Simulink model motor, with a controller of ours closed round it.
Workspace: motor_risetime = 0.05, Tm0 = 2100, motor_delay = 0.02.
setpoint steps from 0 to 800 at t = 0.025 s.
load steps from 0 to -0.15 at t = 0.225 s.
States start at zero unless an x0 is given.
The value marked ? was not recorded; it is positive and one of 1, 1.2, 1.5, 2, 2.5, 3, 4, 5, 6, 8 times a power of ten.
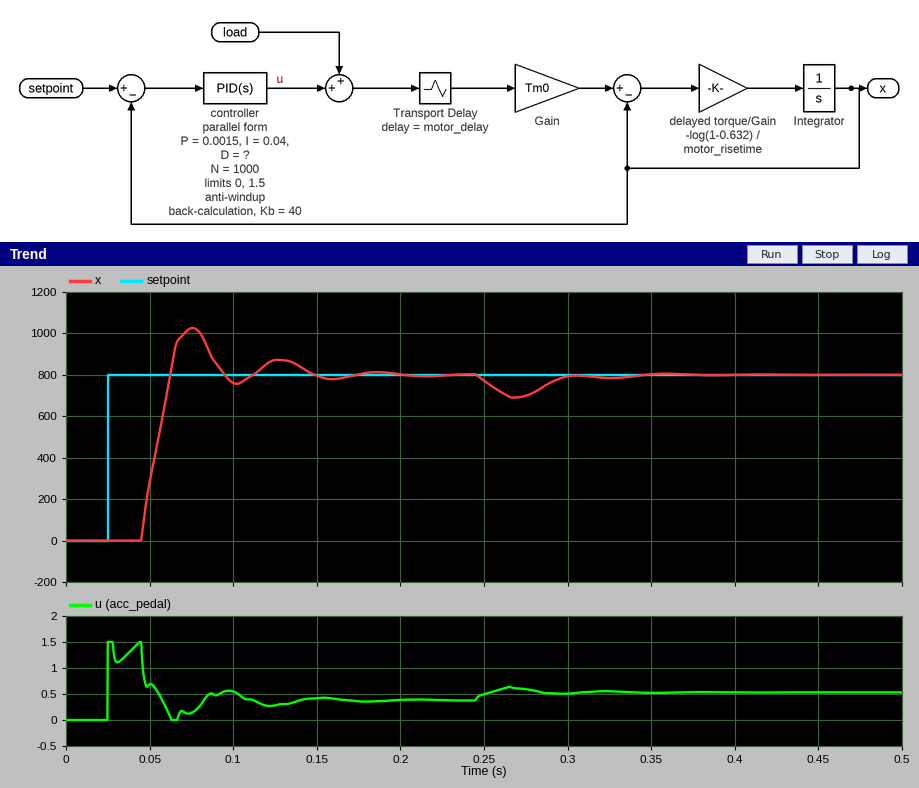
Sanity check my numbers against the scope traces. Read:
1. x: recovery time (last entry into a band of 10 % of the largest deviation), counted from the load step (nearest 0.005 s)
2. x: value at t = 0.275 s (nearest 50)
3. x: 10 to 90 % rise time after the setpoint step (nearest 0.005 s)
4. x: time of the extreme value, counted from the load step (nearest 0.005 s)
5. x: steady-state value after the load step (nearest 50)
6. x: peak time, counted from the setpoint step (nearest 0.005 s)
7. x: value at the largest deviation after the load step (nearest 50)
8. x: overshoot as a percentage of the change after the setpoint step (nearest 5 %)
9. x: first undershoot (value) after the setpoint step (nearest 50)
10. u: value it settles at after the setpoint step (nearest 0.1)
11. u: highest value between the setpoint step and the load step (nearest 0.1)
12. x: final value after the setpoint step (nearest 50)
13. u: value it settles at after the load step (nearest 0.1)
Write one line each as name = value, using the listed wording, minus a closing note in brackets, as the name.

x: recovery time (last entry into a band of 10 % of the largest deviation), counted from the load step = 0.110 s
x: value at t = 0.275 s = 700
x: 10 to 90 % rise time after the setpoint step = 0.015 s
x: time of the extreme value, counted from the load step = 0.045 s
x: steady-state value after the load step = 800
x: peak time, counted from the setpoint step = 0.050 s
x: value at the largest deviation after the load step = 700
x: overshoot as a percentage of the change after the setpoint step = 30 %
x: first undershoot (value) after the setpoint step = 750
u: value it settles at after the setpoint step = 0.4
u: highest value between the setpoint step and the load step = 1.5
x: final value after the setpoint step = 800
u: value it settles at after the load step = 0.5
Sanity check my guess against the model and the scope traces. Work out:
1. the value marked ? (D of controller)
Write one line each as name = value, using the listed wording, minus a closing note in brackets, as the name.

the value marked ? = 1.2e-05
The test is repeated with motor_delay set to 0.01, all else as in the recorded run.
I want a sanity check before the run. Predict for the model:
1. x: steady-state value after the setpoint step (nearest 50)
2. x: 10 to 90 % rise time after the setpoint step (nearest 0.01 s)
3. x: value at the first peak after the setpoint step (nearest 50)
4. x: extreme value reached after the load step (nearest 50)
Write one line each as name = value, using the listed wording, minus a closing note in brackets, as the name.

x: steady-state value after the setpoint step = 800
x: 10 to 90 % rise time after the setpoint step = 0.03 s
x: value at the first peak after the setpoint step = 850
x: extreme value reached after the load step = 750
